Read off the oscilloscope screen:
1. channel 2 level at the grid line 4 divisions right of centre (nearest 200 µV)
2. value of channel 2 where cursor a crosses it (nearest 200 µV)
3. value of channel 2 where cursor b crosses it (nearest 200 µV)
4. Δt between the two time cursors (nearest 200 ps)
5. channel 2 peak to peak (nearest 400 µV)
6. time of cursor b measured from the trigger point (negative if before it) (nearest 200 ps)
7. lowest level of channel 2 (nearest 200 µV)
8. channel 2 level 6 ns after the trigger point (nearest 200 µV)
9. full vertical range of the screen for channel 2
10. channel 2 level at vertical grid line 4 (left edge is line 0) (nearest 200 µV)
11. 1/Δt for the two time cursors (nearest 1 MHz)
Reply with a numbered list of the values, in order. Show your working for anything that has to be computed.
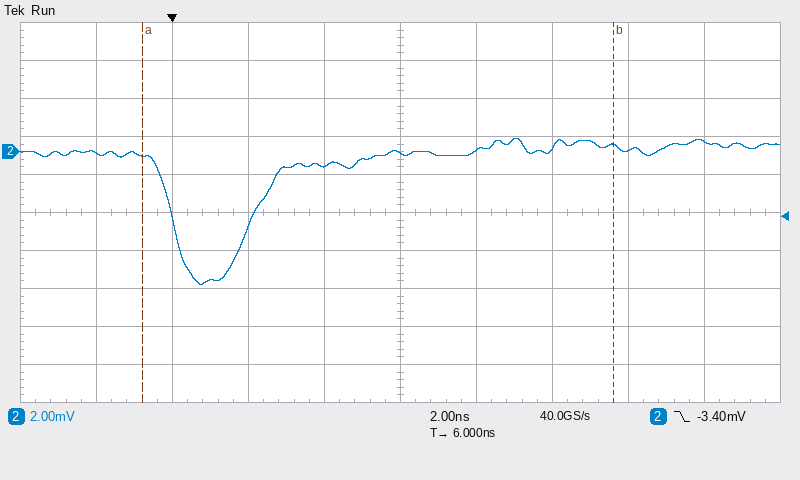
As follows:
1. 600 µV
2. -200 µV
3. 400 µV
4. 12.4 ns
5. 7.6 mV
6. +11.6 ns
7. -7.0 mV
8. 0.0 mV
9. 20 mV
10. -800 µV
11. 1 / 12.4 ns ≈ 81 MHz
